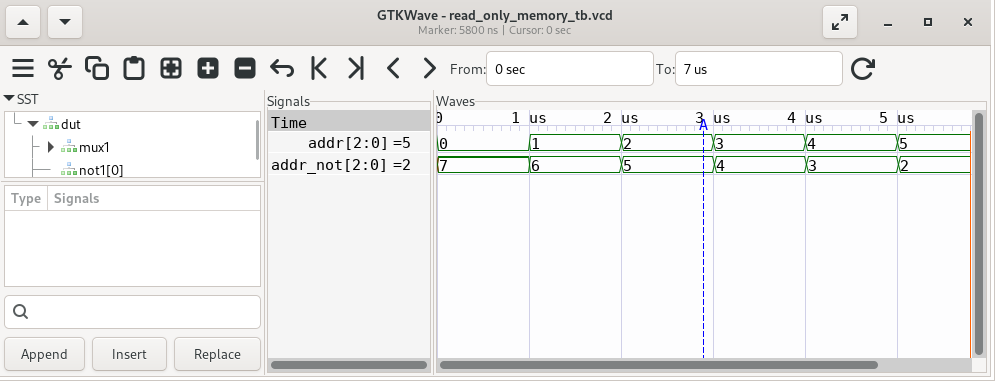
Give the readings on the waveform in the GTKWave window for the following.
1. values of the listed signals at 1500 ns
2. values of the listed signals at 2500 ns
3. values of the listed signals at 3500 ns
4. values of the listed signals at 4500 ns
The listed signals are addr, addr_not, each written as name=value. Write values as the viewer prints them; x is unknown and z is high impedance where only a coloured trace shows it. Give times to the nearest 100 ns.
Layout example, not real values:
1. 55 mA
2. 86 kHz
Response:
1. addr=1, addr_not=6
2. addr=2, addr_not=5
3. addr=3, addr_not=4
4. addr=4, addr_not=3
